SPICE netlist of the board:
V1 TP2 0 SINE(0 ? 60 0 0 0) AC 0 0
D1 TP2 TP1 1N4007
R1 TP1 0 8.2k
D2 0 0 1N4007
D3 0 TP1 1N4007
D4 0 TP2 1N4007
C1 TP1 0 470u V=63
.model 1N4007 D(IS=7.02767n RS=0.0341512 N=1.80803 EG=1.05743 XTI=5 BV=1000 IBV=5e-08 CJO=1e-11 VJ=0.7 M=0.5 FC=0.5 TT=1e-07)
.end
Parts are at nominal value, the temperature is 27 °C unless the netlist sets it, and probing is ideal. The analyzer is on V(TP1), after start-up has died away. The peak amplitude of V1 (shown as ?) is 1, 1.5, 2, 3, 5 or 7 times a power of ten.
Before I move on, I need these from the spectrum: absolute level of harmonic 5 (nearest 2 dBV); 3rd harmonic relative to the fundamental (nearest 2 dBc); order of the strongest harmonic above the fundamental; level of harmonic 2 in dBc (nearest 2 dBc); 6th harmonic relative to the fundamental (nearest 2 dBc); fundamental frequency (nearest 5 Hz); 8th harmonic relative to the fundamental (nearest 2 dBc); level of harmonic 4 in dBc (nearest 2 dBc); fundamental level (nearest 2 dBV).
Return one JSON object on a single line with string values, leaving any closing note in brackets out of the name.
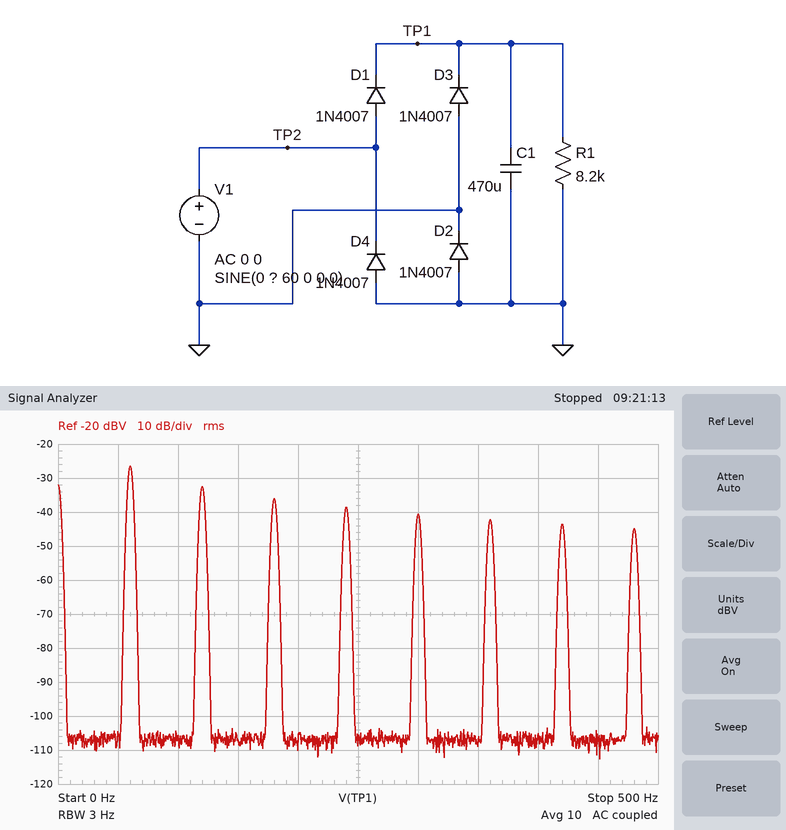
{"absolute level of harmonic 5": "-40 dBV", "3rd harmonic relative to the fundamental": "-10 dBc", "order of the strongest harmonic above the fundamental": "2", "level of harmonic 2 in dBc": "-6 dBc", "6th harmonic relative to the fundamental": "-16 dBc", "fundamental frequency": "60 Hz", "8th harmonic relative to the fundamental": "-18 dBc", "level of harmonic 4 in dBc": "-12 dBc", "fundamental level": "-26 dBV"}
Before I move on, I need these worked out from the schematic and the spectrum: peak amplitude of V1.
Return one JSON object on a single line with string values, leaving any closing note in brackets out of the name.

{"peak amplitude of V1": "50 V"}
